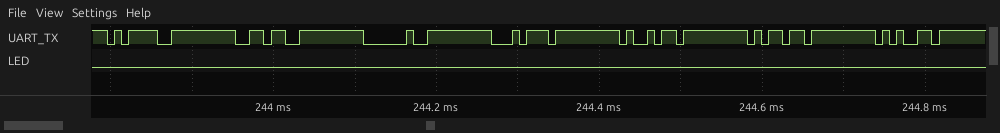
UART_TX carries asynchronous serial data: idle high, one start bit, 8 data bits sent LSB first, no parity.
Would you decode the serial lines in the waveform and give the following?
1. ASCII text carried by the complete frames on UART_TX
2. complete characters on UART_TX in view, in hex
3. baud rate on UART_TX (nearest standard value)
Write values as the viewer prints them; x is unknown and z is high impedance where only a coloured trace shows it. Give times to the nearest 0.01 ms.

"=6 time"
3D, 36, 20, 74, 69, 6D, 65
115200 baud
